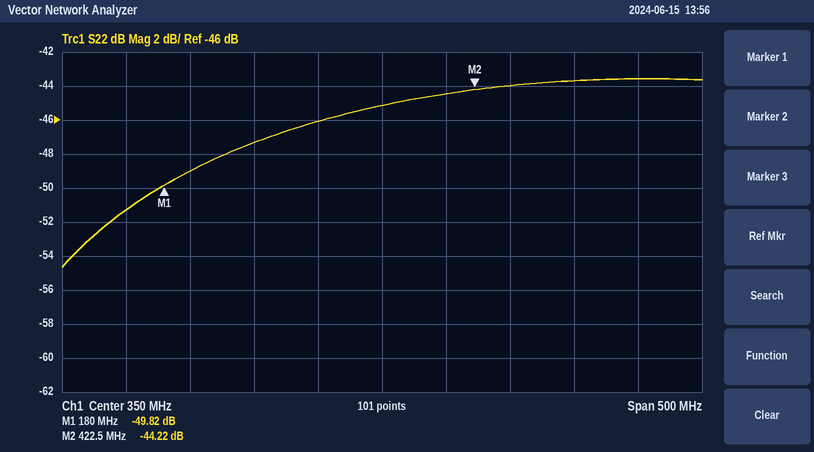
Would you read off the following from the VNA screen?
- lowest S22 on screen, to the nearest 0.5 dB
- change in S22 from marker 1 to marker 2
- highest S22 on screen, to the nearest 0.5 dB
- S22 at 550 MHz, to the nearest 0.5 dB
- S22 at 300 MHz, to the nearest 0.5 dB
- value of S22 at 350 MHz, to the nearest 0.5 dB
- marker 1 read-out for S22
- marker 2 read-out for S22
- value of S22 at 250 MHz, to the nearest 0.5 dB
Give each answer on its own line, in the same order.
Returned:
-54.5 dB
5.60 dB
-43.5 dB
-43.5 dB
-46.0 dB
-45.0 dB
-49.82 dB
-44.22 dB
-47.5 dB
